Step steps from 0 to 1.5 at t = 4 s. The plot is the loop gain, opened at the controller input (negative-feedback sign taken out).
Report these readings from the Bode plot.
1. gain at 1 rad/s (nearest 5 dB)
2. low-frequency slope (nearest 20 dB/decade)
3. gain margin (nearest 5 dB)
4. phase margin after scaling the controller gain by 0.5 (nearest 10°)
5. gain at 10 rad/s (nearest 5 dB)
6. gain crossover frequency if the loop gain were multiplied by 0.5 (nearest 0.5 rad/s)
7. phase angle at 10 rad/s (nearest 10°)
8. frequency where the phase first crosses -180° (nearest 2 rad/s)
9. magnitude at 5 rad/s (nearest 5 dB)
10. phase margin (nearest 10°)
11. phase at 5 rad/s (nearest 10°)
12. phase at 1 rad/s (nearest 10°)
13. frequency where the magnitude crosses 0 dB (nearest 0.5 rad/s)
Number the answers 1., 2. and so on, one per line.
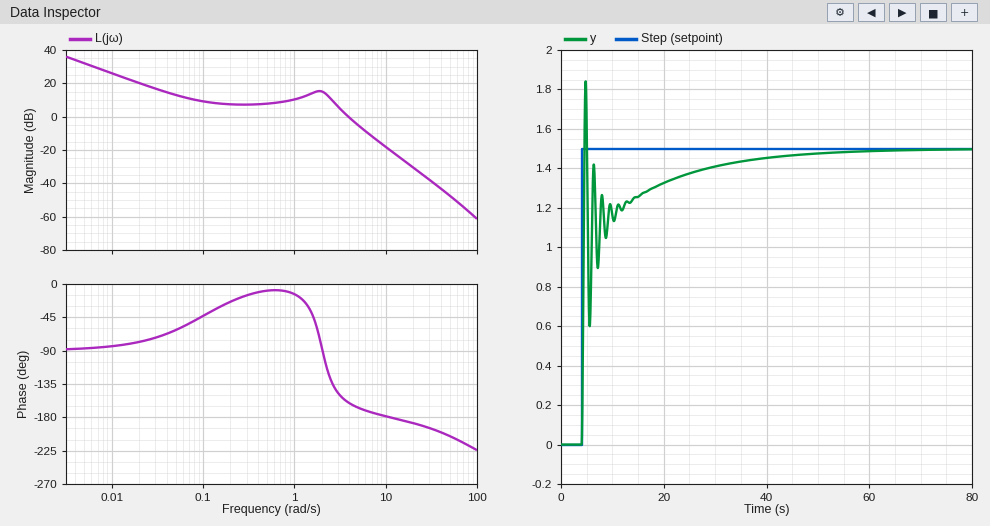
1. 10 dB
2. -20 dB/decade
3. 20 dB
4. 30°
5. -20 dB
6. 3.0 rad/s
7. -180°
8. 12 rad/s
9. -5 dB
10. 20°
11. -170°
12. -10°
13. 4.0 rad/s
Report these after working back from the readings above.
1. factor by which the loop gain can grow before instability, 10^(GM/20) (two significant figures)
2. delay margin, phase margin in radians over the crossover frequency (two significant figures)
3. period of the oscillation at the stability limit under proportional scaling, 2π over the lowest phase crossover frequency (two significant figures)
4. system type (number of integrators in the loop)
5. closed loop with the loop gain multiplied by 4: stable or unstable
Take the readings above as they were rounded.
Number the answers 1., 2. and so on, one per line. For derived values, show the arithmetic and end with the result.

1. 10^(20 / 20) = 10
2. 20 × π / 180 / 4 = 0.087 s
3. 2π / 12 = 0.52 s
4. 1
5. stable
